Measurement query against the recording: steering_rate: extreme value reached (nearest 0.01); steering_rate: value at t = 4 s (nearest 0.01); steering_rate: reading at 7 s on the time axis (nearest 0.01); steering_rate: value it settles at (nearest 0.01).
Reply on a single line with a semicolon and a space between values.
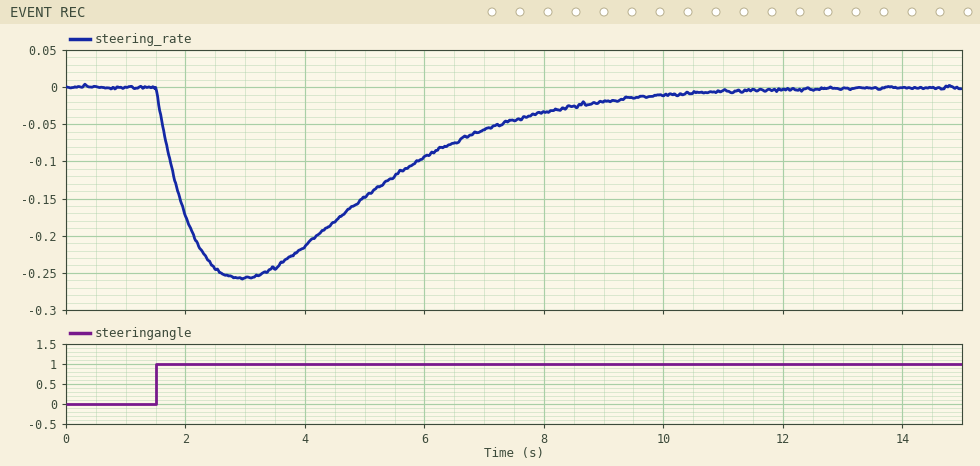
-0.26; -0.21; -0.06; 0.00
